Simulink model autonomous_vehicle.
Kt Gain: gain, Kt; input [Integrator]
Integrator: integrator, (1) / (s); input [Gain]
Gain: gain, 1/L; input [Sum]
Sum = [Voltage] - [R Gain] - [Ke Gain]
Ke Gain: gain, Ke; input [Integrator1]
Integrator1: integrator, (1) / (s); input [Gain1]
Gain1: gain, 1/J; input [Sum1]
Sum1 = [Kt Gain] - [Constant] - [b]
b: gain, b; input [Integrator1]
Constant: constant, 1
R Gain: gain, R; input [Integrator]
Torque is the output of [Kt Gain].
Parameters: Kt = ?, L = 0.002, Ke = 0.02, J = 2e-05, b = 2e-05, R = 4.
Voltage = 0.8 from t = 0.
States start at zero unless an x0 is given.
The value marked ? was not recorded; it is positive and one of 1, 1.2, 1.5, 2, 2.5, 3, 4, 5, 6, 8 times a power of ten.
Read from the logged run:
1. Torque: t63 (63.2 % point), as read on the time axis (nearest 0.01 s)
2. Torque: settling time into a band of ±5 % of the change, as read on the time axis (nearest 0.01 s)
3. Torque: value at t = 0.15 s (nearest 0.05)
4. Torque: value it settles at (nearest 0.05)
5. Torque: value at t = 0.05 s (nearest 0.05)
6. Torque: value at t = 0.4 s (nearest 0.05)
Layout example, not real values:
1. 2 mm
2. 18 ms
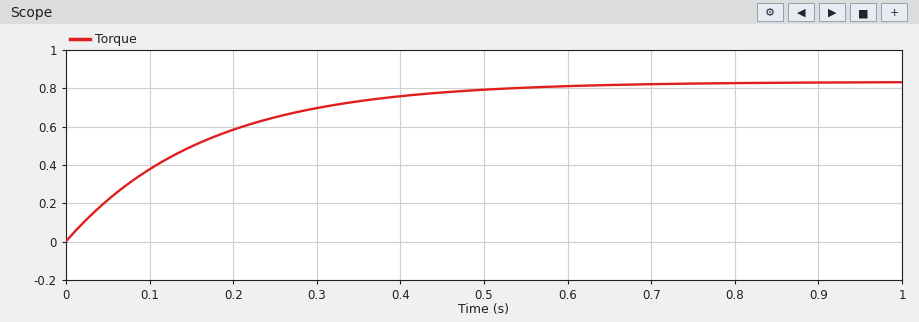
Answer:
1. 0.17 s
2. 0.50 s
3. 0.50
4. 0.85
5. 0.20
6. 0.75
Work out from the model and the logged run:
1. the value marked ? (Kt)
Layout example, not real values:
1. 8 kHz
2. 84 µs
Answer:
1. 0.02
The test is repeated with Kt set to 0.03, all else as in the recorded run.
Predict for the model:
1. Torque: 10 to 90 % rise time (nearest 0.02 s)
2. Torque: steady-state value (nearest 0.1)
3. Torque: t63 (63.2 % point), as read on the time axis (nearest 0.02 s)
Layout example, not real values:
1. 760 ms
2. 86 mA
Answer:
1. 0.26 s
2. 0.9
3. 0.12 s
